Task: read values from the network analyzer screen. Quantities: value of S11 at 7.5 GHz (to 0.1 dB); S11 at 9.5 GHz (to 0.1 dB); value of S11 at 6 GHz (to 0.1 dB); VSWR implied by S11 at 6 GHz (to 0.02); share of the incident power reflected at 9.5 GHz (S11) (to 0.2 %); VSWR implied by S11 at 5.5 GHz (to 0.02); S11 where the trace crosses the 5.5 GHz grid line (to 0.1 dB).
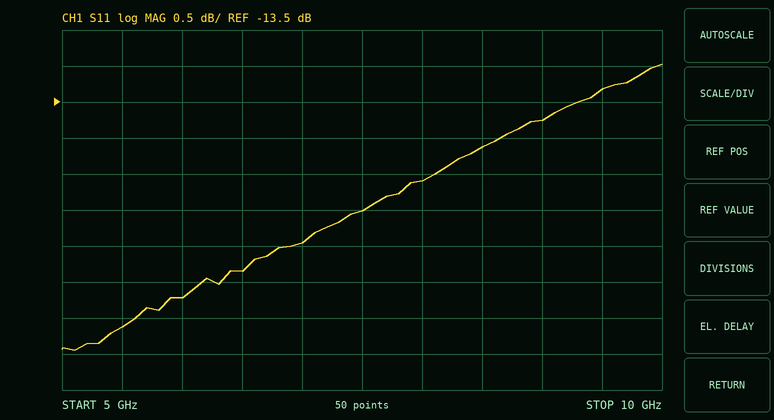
-15.0 dB
-13.3 dB
-16.2 dB
1.36
4.6 %
1.34
-16.6 dB
